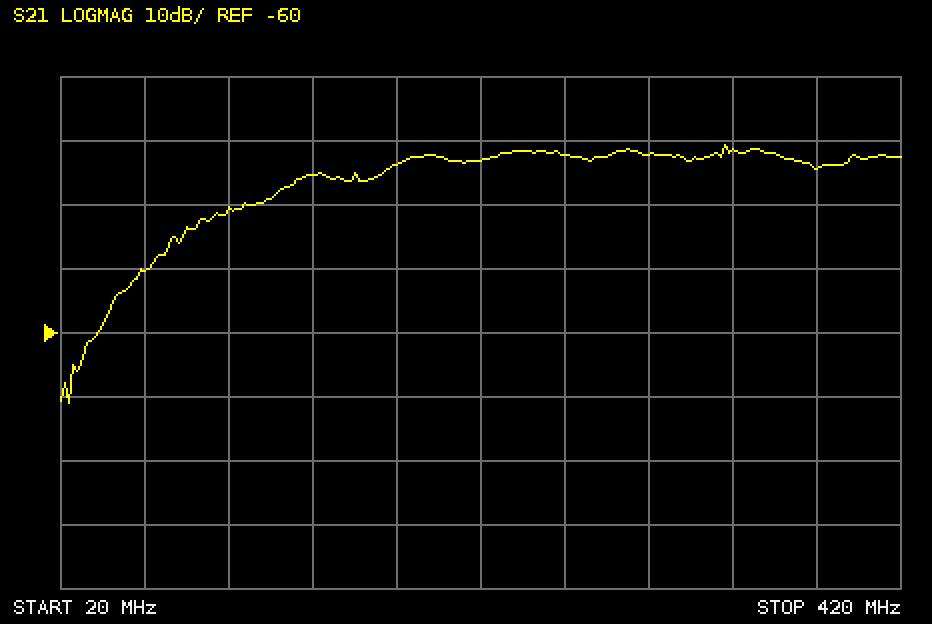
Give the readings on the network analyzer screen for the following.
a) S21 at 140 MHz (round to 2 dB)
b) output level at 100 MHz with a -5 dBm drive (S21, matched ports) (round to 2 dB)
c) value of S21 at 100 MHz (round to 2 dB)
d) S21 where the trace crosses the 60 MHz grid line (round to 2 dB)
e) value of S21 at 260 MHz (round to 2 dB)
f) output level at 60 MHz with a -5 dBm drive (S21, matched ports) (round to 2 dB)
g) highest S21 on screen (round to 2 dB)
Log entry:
-36 dB
-46 dBm
-40 dB
-50 dB
-32 dB
-56 dBm
-30 dB
